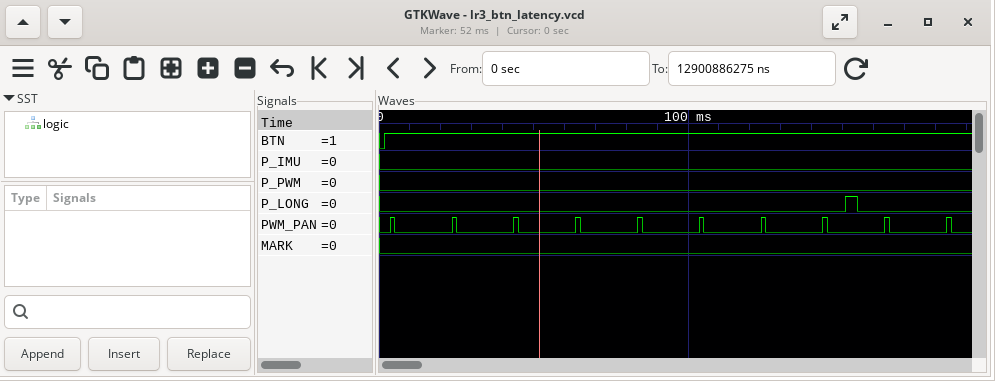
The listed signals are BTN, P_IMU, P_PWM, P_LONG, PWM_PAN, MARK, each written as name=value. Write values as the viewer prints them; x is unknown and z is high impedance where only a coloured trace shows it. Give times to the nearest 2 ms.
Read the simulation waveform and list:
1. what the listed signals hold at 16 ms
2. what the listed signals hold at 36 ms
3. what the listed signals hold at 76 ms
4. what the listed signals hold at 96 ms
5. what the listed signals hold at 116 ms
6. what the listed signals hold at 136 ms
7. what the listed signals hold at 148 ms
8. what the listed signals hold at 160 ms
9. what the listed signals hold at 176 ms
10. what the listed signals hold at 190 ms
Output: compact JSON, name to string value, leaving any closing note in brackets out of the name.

{"what the listed signals hold at 16 ms": "BTN=1, P_IMU=0, P_PWM=0, P_LONG=0, PWM_PAN=0, MARK=0", "what the listed signals hold at 36 ms": "BTN=1, P_IMU=0, P_PWM=0, P_LONG=0, PWM_PAN=0, MARK=0", "what the listed signals hold at 76 ms": "BTN=1, P_IMU=0, P_PWM=0, P_LONG=0, PWM_PAN=0, MARK=0", "what the listed signals hold at 96 ms": "BTN=1, P_IMU=0, P_PWM=0, P_LONG=0, PWM_PAN=0, MARK=0", "what the listed signals hold at 116 ms": "BTN=1, P_IMU=0, P_PWM=0, P_LONG=0, PWM_PAN=0, MARK=0", "what the listed signals hold at 136 ms": "BTN=1, P_IMU=0, P_PWM=0, P_LONG=0, PWM_PAN=0, MARK=0", "what the listed signals hold at 148 ms": "BTN=1, P_IMU=0, P_PWM=0, P_LONG=0, PWM_PAN=0, MARK=0", "what the listed signals hold at 160 ms": "BTN=1, P_IMU=0, P_PWM=0, P_LONG=0, PWM_PAN=0, MARK=0", "what the listed signals hold at 176 ms": "BTN=1, P_IMU=0, P_PWM=0, P_LONG=0, PWM_PAN=0, MARK=0", "what the listed signals hold at 190 ms": "BTN=1, P_IMU=0, P_PWM=0, P_LONG=0, PWM_PAN=0, MARK=0"}
